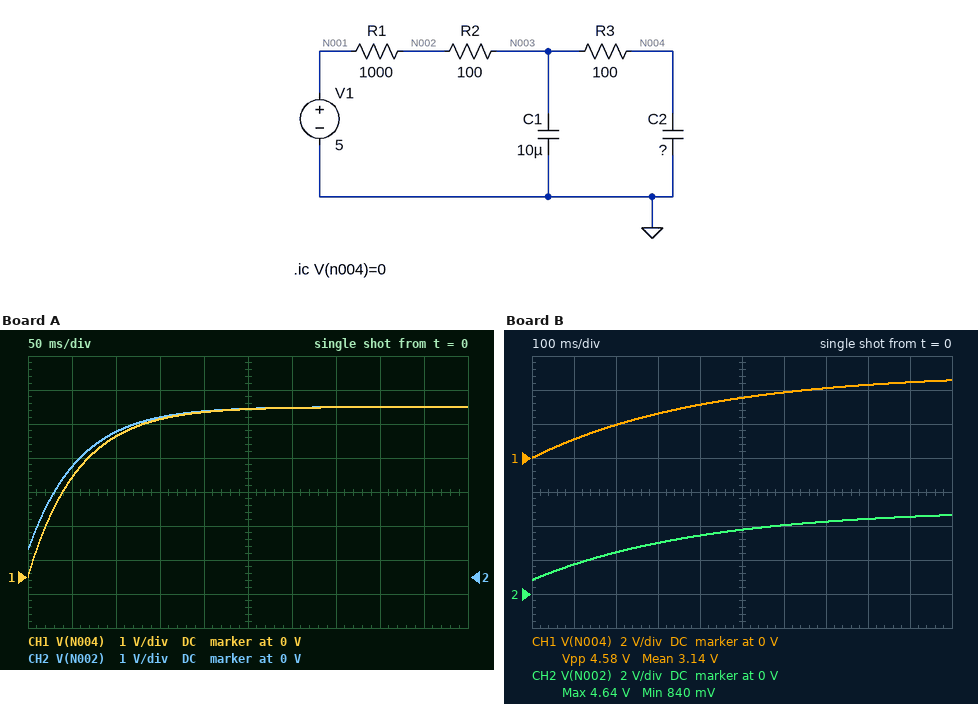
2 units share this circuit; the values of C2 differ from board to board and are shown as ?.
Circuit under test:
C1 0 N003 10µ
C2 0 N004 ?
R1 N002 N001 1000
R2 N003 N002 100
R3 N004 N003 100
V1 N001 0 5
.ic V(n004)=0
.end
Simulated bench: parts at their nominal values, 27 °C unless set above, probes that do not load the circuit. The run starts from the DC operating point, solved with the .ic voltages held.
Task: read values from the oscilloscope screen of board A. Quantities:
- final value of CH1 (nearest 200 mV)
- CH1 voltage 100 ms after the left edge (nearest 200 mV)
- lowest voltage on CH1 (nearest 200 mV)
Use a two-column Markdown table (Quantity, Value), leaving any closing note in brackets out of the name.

| Quantity | Value |
|---|---|
| final value of CH1 | 5.0 V |
| CH1 voltage 100 ms after the left edge | 4.2 V |
| lowest voltage on CH1 | 0 V |
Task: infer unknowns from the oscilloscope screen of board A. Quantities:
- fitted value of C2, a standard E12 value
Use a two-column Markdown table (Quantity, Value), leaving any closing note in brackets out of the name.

| Quantity | Value |
|---|---|
| fitted value of C2, a standard E12 value | 39 µF |
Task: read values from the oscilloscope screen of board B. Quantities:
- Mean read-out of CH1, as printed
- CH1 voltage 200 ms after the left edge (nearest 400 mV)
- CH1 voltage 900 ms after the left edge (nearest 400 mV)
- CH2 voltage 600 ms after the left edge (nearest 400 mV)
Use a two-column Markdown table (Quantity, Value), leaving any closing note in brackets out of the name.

| Quantity | Value |
|---|---|
| Mean read-out of CH1, as printed | 3.14 V |
| CH1 voltage 200 ms after the left edge | 2.0 V |
| CH1 voltage 900 ms after the left edge | 4.4 V |
| CH2 voltage 600 ms after the left edge | 4.0 V |
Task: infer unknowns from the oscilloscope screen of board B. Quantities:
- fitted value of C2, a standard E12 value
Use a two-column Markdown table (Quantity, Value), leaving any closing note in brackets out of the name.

| Quantity | Value |
|---|---|
| fitted value of C2, a standard E12 value | 330 µF |
